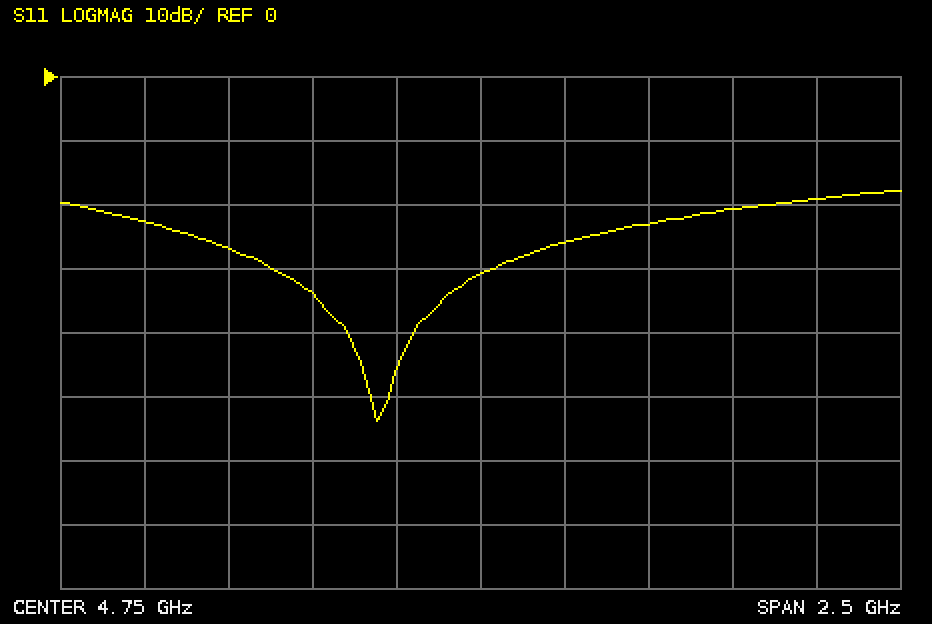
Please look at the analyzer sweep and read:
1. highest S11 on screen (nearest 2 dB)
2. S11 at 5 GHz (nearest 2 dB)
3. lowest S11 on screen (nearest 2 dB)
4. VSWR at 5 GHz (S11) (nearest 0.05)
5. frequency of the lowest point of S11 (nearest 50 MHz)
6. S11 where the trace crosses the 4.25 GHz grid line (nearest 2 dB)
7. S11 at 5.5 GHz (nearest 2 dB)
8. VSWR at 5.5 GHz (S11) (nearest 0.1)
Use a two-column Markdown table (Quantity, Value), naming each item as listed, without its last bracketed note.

| Quantity | Value |
|---|---|
| highest S11 on screen | -18 dB |
| S11 at 5 GHz | -26 dB |
| lowest S11 on screen | -54 dB |
| VSWR at 5 GHz (S11) | 1.10 |
| frequency of the lowest point of S11 | 4.45 GHz |
| S11 where the trace crosses the 4.25 GHz grid line | -34 dB |
| S11 at 5.5 GHz | -20 dB |
| VSWR at 5.5 GHz (S11) | 1.2 |
